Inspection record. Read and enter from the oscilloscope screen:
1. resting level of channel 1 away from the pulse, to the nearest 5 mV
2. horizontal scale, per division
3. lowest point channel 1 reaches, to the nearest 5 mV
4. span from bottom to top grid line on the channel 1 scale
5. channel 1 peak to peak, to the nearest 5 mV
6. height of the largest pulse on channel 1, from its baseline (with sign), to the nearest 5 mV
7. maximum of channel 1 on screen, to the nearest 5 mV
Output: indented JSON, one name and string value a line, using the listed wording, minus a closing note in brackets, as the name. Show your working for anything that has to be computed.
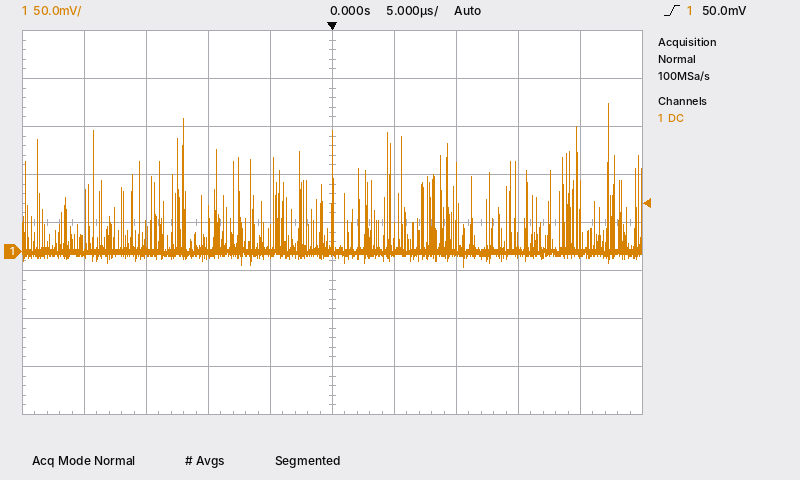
{
  "resting level of channel 1 away from the pulse, to the nearest 5 mV": "0 mV",
  "horizontal scale, per division": "5 µs",
  "lowest point channel 1 reaches, to the nearest 5 mV": "-15 mV",
  "span from bottom to top grid line on the channel 1 scale": "400 mV",
  "channel 1 peak to peak, to the nearest 5 mV": "155 mV − (-15 mV) = 170 mV",
  "height of the largest pulse on channel 1, from its baseline (with sign), to the nearest 5 mV": "155 mV − (0 mV) = +155 mV",
  "maximum of channel 1 on screen, to the nearest 5 mV": "155 mV"
}
